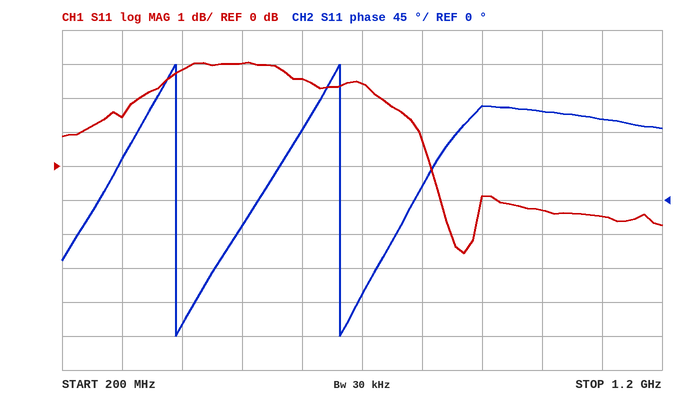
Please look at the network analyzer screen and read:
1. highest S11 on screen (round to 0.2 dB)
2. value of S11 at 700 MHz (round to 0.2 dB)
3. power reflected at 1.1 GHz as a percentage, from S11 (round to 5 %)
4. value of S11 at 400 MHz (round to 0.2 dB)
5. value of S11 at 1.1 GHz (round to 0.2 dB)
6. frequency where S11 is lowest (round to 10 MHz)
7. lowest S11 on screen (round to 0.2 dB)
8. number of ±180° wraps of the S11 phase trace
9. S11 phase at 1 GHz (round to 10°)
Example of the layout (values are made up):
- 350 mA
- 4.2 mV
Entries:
- 3.0 dB
- 2.4 dB
- 70 %
- 2.8 dB
- -1.4 dB
- 870 MHz
- -2.6 dB
- 2
- 120°
